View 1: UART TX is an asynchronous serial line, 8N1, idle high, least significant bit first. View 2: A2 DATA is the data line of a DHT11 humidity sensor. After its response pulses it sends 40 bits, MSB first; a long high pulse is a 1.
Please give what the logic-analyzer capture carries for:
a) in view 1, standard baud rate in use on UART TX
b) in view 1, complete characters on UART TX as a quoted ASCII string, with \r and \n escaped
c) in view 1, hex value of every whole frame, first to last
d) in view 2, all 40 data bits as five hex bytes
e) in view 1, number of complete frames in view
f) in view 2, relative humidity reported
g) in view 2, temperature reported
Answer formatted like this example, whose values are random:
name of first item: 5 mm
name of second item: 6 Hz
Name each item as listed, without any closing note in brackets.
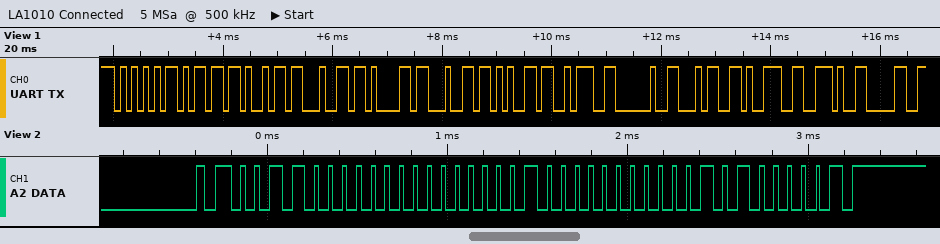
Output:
in view 1, standard baud rate in use on UART TX: 9600 baud
in view 1, complete characters on UART TX as a quoted ASCII string, with \r and \n escaped: "Umidade: 49.0"
in view 1, hex value of every whole frame, first to last: 55 6D 69 64 61 64 65 3A 20 34 39 2E 30
in view 2, all 40 data bits as five hex bytes: 30 00 10 01 41
in view 1, number of complete frames in view: 13
in view 2, relative humidity reported: 48 %
in view 2, temperature reported: 16.1 °C
